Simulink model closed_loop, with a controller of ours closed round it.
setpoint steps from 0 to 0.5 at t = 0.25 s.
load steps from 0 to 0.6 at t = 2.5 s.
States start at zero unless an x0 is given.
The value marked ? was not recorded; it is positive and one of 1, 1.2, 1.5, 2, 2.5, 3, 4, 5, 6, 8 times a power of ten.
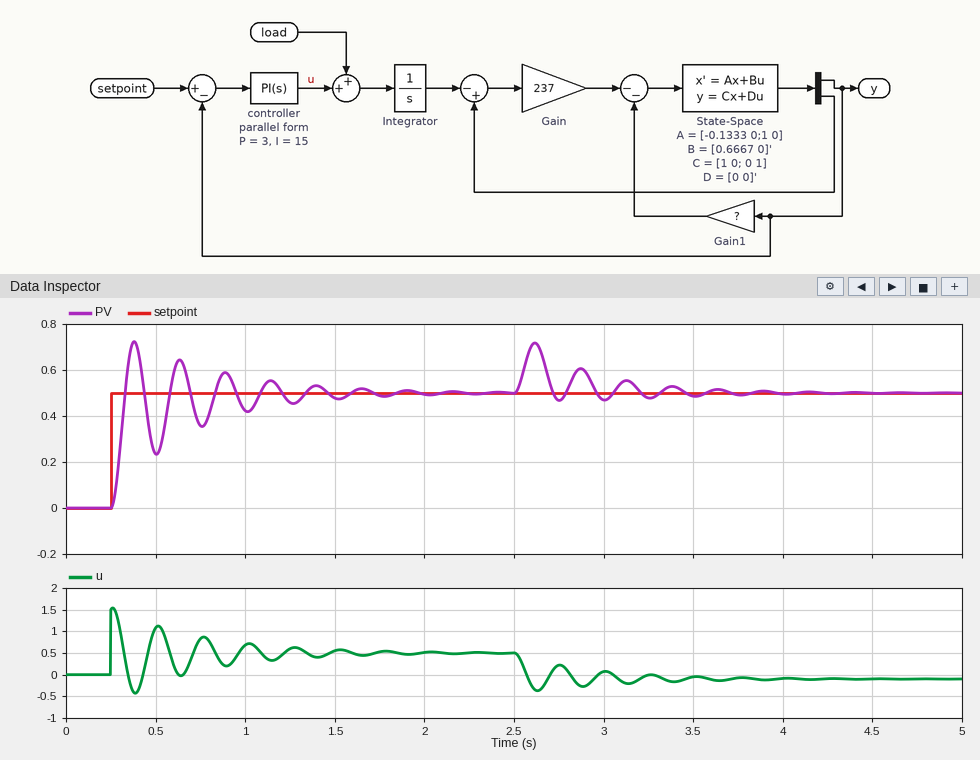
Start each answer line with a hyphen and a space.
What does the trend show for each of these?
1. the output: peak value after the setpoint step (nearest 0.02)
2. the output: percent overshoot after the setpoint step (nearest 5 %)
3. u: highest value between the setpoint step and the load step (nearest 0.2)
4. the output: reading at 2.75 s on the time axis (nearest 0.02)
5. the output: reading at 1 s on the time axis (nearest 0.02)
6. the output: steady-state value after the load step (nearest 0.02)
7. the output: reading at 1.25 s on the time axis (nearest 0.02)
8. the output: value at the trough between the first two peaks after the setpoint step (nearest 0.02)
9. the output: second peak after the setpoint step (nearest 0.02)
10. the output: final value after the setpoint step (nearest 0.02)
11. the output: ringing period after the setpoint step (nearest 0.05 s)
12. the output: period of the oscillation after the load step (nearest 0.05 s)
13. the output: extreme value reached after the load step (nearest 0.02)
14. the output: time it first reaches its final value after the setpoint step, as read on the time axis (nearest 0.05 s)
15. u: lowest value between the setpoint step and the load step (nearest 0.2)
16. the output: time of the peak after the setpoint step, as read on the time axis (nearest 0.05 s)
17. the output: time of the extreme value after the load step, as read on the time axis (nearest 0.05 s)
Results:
- 0.72
- 45 %
- 1.6
- 0.46
- 0.42
- 0.50
- 0.46
- 0.24
- 0.64
- 0.50
- 0.25 s
- 0.25 s
- 0.72
- 0.35 s
- -0.4
- 0.40 s
- 2.60 s
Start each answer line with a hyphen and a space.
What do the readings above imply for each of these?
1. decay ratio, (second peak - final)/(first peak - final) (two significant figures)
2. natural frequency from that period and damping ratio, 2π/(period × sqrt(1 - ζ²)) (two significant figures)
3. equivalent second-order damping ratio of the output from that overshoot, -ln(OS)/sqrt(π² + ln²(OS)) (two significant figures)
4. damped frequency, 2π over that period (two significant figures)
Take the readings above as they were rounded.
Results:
- 0.64
- 26 rad/s
- 0.25
- 25 rad/s
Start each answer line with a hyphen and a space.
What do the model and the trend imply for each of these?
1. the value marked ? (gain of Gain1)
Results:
- 12
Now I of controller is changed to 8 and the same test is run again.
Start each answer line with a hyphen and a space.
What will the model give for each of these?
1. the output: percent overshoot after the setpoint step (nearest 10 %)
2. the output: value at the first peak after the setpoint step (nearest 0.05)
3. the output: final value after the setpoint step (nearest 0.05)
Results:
- 30 %
- 0.65
- 0.50
